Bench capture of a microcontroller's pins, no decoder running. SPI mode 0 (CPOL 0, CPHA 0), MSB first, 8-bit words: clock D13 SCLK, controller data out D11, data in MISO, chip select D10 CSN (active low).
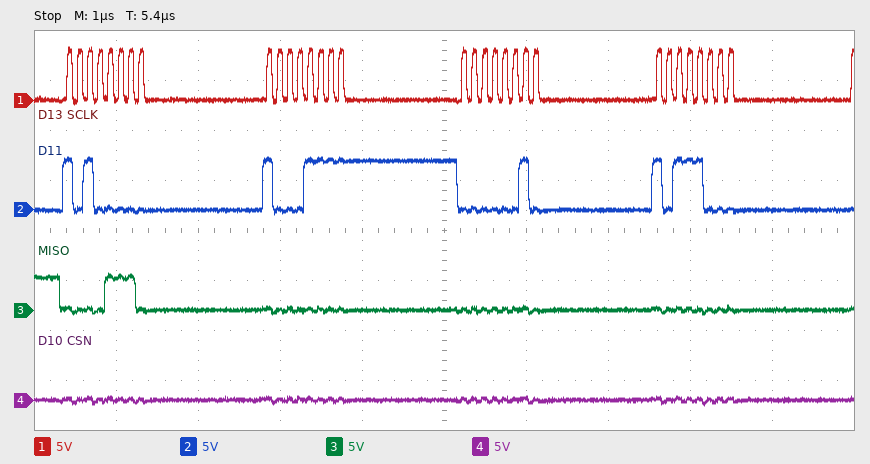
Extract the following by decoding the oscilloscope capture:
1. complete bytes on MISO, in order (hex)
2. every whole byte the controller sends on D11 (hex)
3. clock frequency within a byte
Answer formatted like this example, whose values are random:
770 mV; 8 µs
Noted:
0E 00 00 00; A0 8F 02 B8; 8 MHz
